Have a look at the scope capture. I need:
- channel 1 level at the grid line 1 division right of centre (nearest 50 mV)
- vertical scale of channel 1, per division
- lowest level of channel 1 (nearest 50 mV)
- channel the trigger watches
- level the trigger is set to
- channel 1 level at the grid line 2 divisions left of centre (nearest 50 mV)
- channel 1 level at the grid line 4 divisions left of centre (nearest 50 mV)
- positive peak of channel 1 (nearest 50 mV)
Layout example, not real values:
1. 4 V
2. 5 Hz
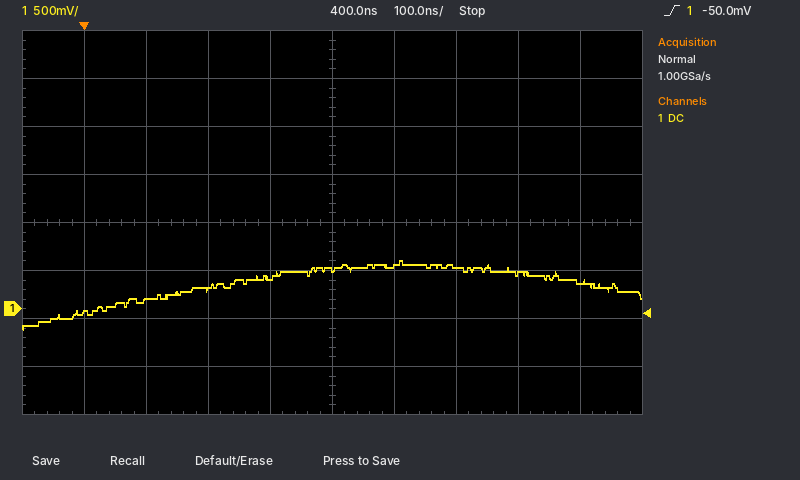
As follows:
1. 450 mV
2. 500 mV
3. -200 mV
4. channel 1
5. -50.0 mV
6. 200 mV
7. -50 mV
8. 500 mV
